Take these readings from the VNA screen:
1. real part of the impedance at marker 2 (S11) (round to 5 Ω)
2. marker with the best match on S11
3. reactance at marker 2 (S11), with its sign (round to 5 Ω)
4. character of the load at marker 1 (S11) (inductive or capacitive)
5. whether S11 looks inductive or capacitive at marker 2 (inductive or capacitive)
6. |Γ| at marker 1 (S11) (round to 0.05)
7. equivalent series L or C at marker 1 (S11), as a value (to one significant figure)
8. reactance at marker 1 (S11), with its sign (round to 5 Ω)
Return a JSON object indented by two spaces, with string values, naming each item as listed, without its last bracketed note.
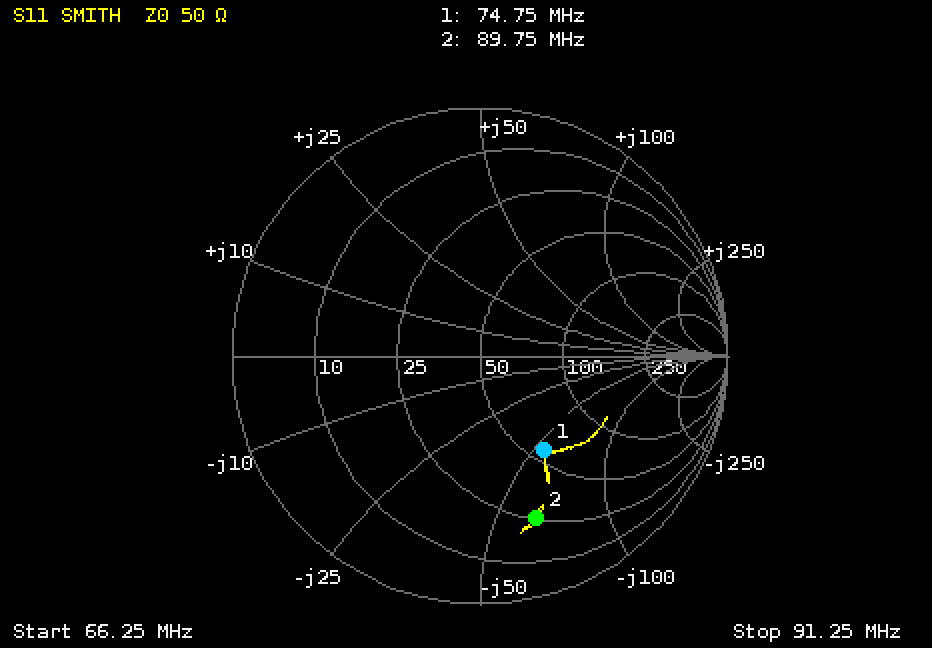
{
  "real part of the impedance at marker 2 (S11)": "25 Ω",
  "marker with the best match on S11": "marker 1",
  "reactance at marker 2 (S11), with its sign": "-65 Ω",
  "character of the load at marker 1 (S11)": "capacitive",
  "whether S11 looks inductive or capacitive at marker 2": "capacitive",
  "|Γ| at marker 1 (S11)": "0.45",
  "equivalent series L or C at marker 1 (S11), as a value": "40 pF",
  "reactance at marker 1 (S11), with its sign": "-55 Ω"
}
